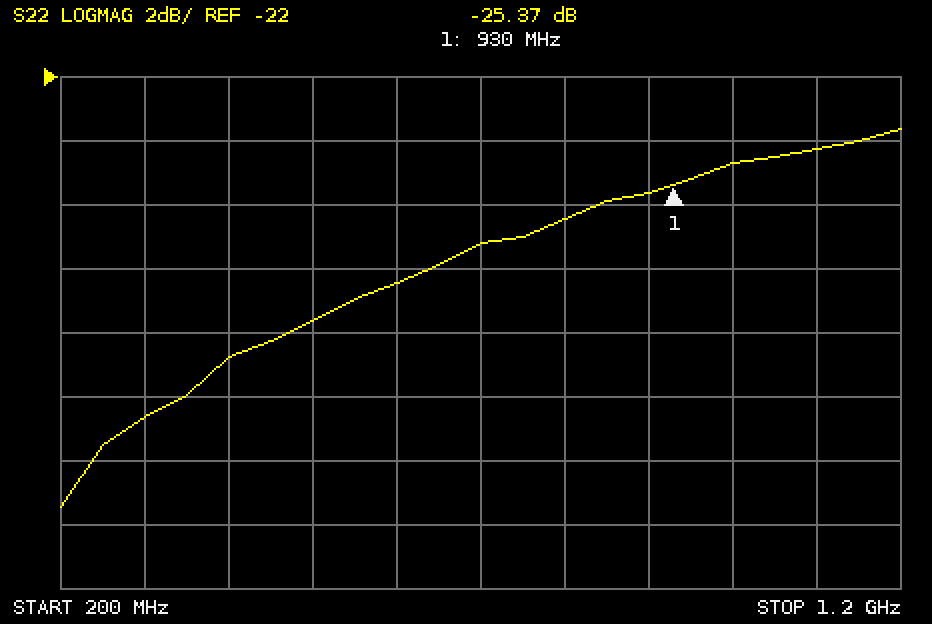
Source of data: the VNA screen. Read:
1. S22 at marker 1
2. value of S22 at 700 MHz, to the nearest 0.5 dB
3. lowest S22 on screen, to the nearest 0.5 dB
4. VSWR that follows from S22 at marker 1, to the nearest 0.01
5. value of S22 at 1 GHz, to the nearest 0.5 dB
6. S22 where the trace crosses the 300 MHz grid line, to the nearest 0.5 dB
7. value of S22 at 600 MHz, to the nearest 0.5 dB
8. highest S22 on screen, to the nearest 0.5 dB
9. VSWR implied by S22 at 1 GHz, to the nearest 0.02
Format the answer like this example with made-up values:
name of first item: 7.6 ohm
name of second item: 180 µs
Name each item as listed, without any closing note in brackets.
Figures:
S22 at marker 1: -25.37 dB
value of S22 at 700 MHz, to the nearest 0.5 dB: -27.0 dB
lowest S22 on screen, to the nearest 0.5 dB: -35.5 dB
VSWR that follows from S22 at marker 1, to the nearest 0.01: 1.11
value of S22 at 1 GHz, to the nearest 0.5 dB: -24.5 dB
S22 where the trace crosses the 300 MHz grid line, to the nearest 0.5 dB: -32.5 dB
value of S22 at 600 MHz, to the nearest 0.5 dB: -28.5 dB
highest S22 on screen, to the nearest 0.5 dB: -23.5 dB
VSWR implied by S22 at 1 GHz, to the nearest 0.02: 1.12
